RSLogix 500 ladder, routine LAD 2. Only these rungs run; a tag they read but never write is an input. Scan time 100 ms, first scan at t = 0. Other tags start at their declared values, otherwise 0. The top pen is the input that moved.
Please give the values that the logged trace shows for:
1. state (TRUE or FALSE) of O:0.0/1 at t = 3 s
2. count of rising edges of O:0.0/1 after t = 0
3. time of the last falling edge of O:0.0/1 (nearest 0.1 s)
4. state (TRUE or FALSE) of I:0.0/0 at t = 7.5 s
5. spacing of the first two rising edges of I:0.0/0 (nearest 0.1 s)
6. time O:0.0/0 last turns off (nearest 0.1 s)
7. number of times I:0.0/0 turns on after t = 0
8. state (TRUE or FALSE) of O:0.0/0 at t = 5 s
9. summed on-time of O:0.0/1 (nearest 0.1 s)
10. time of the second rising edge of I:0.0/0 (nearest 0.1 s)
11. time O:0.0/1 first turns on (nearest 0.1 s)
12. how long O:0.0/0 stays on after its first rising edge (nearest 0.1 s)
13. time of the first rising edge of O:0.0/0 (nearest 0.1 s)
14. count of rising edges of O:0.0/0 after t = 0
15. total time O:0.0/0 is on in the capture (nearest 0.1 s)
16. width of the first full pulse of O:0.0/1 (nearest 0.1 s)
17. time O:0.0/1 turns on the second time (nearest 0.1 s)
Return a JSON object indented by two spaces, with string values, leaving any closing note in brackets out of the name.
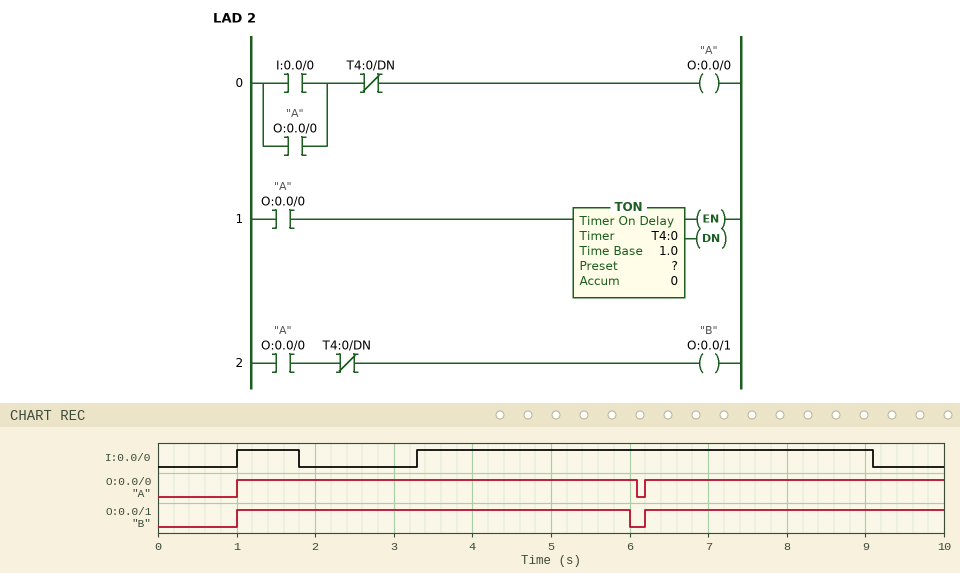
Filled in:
{
  "state (TRUE or FALSE) of O:0.0/1 at t = 3 s": "TRUE",
  "count of rising edges of O:0.0/1 after t = 0": "2",
  "time of the last falling edge of O:0.0/1": "6.0 s",
  "state (TRUE or FALSE) of I:0.0/0 at t = 7.5 s": "TRUE",
  "spacing of the first two rising edges of I:0.0/0": "2.3 s",
  "time O:0.0/0 last turns off": "6.1 s",
  "number of times I:0.0/0 turns on after t = 0": "2",
  "state (TRUE or FALSE) of O:0.0/0 at t = 5 s": "TRUE",
  "summed on-time of O:0.0/1": "8.8 s",
  "time of the second rising edge of I:0.0/0": "3.3 s",
  "time O:0.0/1 first turns on": "1.0 s",
  "how long O:0.0/0 stays on after its first rising edge": "5.1 s",
  "time of the first rising edge of O:0.0/0": "1.0 s",
  "count of rising edges of O:0.0/0 after t = 0": "2",
  "total time O:0.0/0 is on in the capture": "8.9 s",
  "width of the first full pulse of O:0.0/1": "5.0 s",
  "time O:0.0/1 turns on the second time": "6.2 s"
}
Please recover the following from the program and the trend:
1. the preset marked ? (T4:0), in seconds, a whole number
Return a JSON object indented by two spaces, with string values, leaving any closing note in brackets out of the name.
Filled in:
{
  "the preset marked ? (T4:0), in seconds, a whole number": "5 s"
}
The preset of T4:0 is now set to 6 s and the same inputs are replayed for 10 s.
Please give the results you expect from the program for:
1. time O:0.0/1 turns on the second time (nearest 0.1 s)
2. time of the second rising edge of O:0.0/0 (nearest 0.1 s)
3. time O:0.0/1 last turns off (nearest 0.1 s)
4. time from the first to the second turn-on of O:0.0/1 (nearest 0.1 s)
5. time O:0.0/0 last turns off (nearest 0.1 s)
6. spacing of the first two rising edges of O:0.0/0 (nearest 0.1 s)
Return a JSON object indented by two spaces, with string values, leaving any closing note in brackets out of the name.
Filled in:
{
  "time O:0.0/1 turns on the second time": "7.2 s",
  "time of the second rising edge of O:0.0/0": "7.2 s",
  "time O:0.0/1 last turns off": "7.0 s",
  "time from the first to the second turn-on of O:0.0/1": "6.2 s",
  "time O:0.0/0 last turns off": "7.1 s",
  "spacing of the first two rising edges of O:0.0/0": "6.2 s"
}
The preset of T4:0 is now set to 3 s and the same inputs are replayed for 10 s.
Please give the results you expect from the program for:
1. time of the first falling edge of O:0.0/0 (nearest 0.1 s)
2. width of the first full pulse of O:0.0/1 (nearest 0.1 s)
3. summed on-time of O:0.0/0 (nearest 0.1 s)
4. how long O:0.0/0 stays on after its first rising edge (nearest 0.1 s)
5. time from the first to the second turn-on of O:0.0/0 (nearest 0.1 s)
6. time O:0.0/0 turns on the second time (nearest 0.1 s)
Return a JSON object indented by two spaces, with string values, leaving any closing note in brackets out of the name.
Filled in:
{
  "time of the first falling edge of O:0.0/0": "4.1 s",
  "width of the first full pulse of O:0.0/1": "3.0 s",
  "summed on-time of O:0.0/0": "8.8 s",
  "how long O:0.0/0 stays on after its first rising edge": "3.1 s",
  "time from the first to the second turn-on of O:0.0/0": "3.2 s",
  "time O:0.0/0 turns on the second time": "4.2 s"
}
